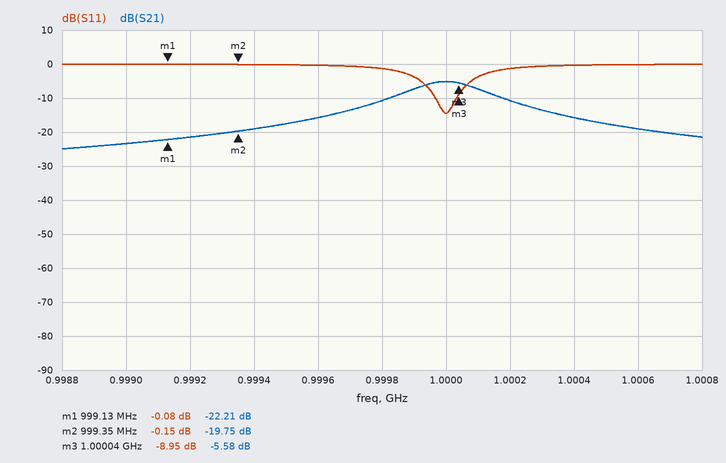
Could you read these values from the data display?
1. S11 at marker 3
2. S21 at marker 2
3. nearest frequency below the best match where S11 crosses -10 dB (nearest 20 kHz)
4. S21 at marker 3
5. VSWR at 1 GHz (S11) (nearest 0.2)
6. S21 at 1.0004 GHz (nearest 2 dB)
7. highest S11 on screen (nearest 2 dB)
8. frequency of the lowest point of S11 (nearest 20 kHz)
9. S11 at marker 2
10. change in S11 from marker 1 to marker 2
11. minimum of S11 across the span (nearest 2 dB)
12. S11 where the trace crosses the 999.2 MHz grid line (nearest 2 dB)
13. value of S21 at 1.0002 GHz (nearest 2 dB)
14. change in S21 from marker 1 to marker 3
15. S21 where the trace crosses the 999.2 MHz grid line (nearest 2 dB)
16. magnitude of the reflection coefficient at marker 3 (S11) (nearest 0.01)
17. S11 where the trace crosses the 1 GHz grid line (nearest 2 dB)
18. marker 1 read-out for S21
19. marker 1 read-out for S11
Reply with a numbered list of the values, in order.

1. -8.95 dB
2. -19.75 dB
3. 999.96 MHz
4. -5.58 dB
5. 1.4
6. -16 dB
7. 0 dB
8. 1.00000 GHz
9. -0.15 dB
10. -0.07 dB
11. -14 dB
12. 0 dB
13. -10 dB
14. 16.63 dB
15. -22 dB
16. 0.36
17. -14 dB
18. -22.21 dB
19. -0.08 dB
